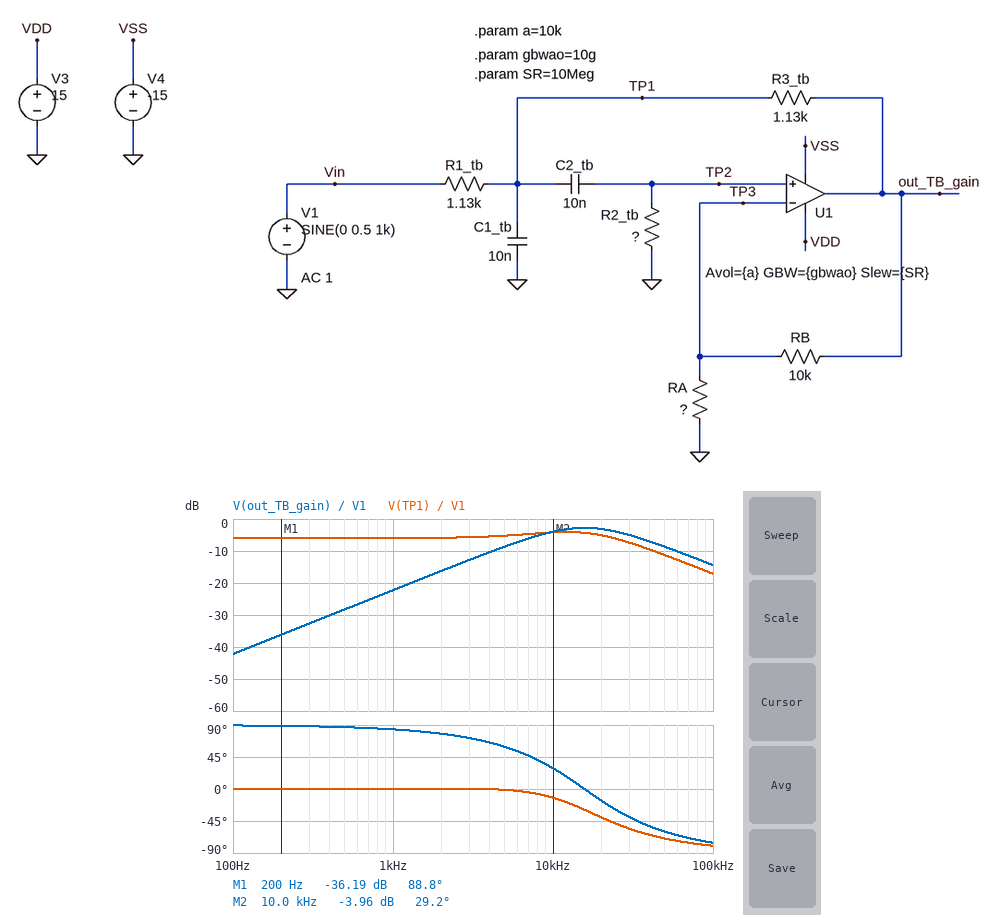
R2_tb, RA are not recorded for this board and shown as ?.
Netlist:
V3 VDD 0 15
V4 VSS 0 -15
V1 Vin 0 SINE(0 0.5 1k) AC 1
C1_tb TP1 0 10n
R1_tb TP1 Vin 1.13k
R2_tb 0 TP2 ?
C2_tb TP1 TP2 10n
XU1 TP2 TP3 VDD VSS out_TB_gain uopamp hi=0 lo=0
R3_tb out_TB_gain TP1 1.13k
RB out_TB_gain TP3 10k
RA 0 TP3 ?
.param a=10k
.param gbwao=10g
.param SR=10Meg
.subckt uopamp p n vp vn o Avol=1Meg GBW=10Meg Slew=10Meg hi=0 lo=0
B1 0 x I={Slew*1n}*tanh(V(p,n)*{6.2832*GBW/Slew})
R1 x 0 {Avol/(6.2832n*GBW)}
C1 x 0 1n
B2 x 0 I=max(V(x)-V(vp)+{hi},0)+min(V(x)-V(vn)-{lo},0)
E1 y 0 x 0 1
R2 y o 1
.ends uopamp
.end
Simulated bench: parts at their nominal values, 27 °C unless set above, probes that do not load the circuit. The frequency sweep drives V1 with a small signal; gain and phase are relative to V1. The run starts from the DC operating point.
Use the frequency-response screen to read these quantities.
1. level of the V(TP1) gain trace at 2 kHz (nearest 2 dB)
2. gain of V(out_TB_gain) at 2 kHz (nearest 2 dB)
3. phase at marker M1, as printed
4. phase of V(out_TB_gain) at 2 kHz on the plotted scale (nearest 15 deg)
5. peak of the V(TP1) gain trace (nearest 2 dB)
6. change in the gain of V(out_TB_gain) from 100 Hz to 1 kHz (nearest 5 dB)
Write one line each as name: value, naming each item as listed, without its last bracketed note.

level of the V(TP1) gain trace at 2 kHz: -6 dB
gain of V(out_TB_gain) at 2 kHz: -16 dB
phase at marker M1, as printed: 88.8 deg
phase of V(out_TB_gain) at 2 kHz on the plotted scale: 75 deg
peak of the V(TP1) gain trace: -4 dB
change in the gain of V(out_TB_gain) from 100 Hz to 1 kHz: 20 dB
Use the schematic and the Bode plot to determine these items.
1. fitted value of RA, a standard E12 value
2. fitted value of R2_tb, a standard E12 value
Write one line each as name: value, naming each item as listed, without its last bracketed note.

fitted value of RA, a standard E12 value: 27 kΩ
fitted value of R2_tb, a standard E12 value: 1.8 kΩ
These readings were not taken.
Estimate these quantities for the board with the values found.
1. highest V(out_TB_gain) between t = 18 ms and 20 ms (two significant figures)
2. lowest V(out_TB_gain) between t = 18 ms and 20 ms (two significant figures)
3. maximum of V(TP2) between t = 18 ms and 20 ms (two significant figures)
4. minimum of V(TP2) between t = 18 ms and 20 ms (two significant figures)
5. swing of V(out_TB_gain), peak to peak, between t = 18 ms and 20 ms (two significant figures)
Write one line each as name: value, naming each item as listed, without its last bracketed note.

highest V(out_TB_gain) between t = 18 ms and 20 ms: 39 mV
lowest V(out_TB_gain) between t = 18 ms and 20 ms: -39 mV
maximum of V(TP2) between t = 18 ms and 20 ms: 28 mV
minimum of V(TP2) between t = 18 ms and 20 ms: -28 mV
swing of V(out_TB_gain), peak to peak, between t = 18 ms and 20 ms: 77 mV
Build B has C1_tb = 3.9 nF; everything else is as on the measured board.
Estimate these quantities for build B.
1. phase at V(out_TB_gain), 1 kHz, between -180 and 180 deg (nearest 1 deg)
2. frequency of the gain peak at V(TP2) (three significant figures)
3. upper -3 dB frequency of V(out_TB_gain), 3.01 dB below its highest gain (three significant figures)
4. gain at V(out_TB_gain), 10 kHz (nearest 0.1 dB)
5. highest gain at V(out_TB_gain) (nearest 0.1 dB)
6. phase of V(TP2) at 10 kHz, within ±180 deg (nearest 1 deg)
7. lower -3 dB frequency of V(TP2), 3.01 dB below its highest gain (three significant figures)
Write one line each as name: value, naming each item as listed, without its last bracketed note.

phase at V(out_TB_gain), 1 kHz, between -180 and 180 deg: 85 deg
frequency of the gain peak at V(TP2): 25.2 kHz
upper -3 dB frequency of V(out_TB_gain), 3.01 dB below its highest gain: 63.8 kHz
gain at V(out_TB_gain), 10 kHz: -3.8 dB
highest gain at V(out_TB_gain): -0.8 dB
phase of V(TP2) at 10 kHz, within ±180 deg: 45 deg
lower -3 dB frequency of V(TP2), 3.01 dB below its highest gain: 9.94 kHz
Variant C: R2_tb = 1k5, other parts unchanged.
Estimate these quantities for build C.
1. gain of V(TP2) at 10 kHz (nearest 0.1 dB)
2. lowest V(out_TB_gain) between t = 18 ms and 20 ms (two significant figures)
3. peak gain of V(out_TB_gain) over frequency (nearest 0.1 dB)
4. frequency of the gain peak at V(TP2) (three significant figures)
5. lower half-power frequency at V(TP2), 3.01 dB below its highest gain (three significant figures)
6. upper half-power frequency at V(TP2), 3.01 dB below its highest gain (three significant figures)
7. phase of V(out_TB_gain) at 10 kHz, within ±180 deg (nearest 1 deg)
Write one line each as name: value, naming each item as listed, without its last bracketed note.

gain of V(TP2) at 10 kHz: -8.2 dB
lowest V(out_TB_gain) between t = 18 ms and 20 ms: -32 mV
peak gain of V(out_TB_gain) over frequency: -3.9 dB
frequency of the gain peak at V(TP2): 17.3 kHz
lower half-power frequency at V(TP2), 3.01 dB below its highest gain: 7.87 kHz
upper half-power frequency at V(TP2), 3.01 dB below its highest gain: 37.9 kHz
phase of V(out_TB_gain) at 10 kHz, within ±180 deg: 33 deg
